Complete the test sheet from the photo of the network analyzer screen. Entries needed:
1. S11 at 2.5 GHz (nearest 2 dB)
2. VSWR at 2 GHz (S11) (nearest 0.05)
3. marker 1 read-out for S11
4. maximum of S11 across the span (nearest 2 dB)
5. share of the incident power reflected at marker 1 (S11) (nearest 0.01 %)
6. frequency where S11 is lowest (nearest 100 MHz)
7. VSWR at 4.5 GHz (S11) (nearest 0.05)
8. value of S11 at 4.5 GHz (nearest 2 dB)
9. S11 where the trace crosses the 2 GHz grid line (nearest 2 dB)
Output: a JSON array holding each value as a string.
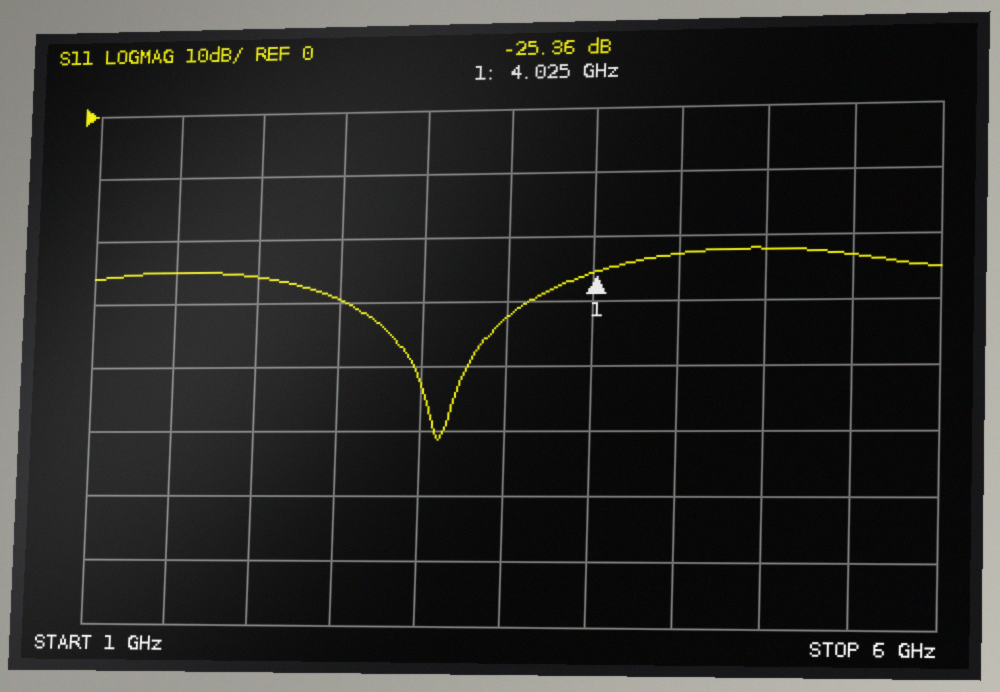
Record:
["-30 dB", "1.10", "-25.36 dB", "-22 dB", "0.29 %", "3.1 GHz", "1.15", "-22 dB", "-26 dB"]
